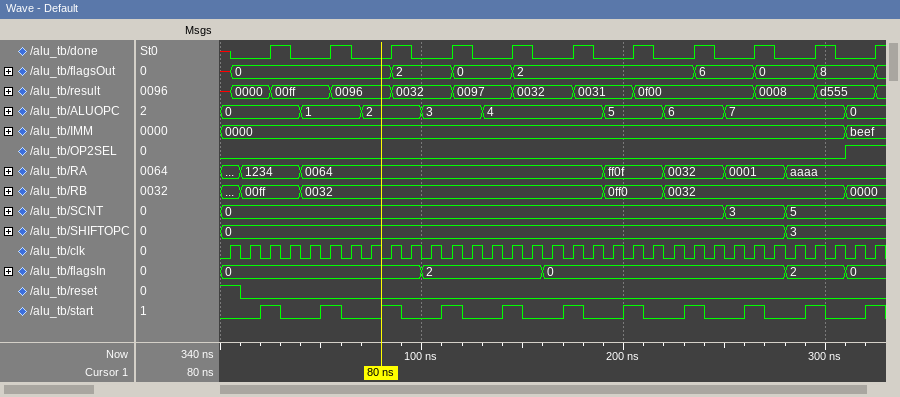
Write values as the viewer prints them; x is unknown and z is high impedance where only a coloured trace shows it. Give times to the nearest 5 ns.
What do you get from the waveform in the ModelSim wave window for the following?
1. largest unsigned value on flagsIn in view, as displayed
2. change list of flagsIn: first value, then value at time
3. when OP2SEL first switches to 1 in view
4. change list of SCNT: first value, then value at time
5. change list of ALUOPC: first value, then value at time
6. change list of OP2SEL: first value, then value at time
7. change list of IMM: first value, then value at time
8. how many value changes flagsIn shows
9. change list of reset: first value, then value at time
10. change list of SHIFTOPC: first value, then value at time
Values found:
2
0, 2 at 100 ns, 0 at 160 ns, 2 at 280 ns, 0 at 310 ns
310 ns
0, 3 at 250 ns, 5 at 280 ns
0, 1 at 40 ns, 2 at 70 ns, 3 at 100 ns, 4 at 130 ns, 5 at 190 ns, 6 at 220 ns, 7 at 250 ns, 0 at 310 ns
0, 1 at 310 ns
0000, beef at 310 ns
4
1, 0 at 10 ns
0, 3 at 280 ns
